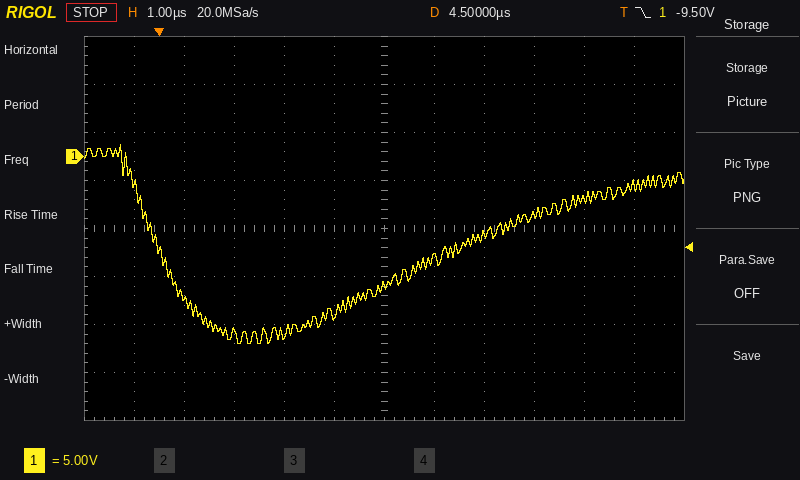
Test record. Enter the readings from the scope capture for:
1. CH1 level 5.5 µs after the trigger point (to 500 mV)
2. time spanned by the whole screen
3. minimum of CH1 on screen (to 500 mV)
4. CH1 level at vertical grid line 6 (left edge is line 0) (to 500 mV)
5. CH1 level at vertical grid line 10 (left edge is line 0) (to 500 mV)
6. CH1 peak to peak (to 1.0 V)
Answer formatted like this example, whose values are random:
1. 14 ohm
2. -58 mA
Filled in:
1. -10.5 V
2. 12 µs
3. -19.5 V
4. -13.5 V
5. -4.5 V
6. 21.0 V
